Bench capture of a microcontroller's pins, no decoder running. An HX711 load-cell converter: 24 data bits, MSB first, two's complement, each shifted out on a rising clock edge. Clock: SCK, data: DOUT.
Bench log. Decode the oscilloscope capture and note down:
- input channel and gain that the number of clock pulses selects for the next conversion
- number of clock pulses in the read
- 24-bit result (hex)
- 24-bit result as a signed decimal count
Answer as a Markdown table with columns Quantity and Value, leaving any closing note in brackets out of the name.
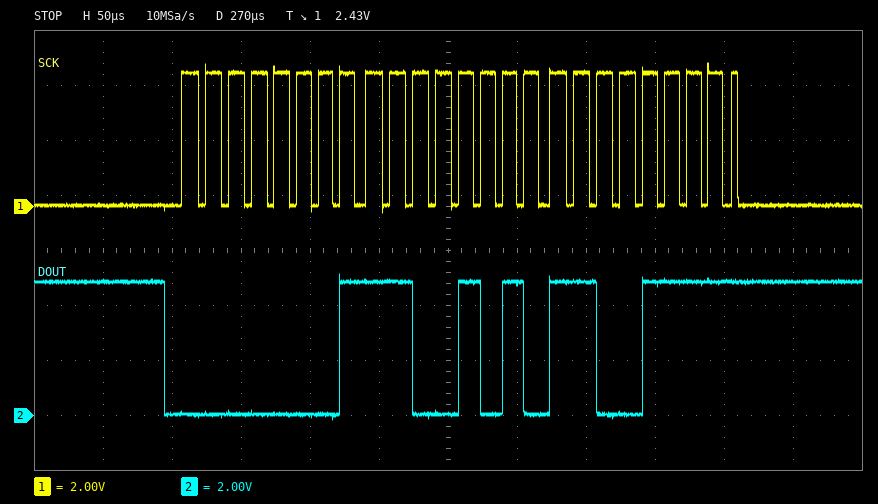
| Quantity | Value |
|---|---|
| input channel and gain that the number of clock pulses selects for the next conversion | channel A, gain 128 |
| number of clock pulses in the read | 25 |
| 24-bit result | 0x01CACF |
| 24-bit result as a signed decimal count | 117455 |
